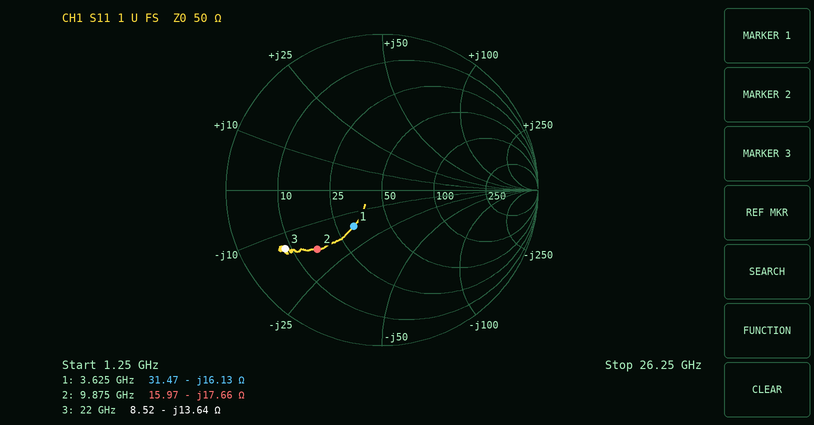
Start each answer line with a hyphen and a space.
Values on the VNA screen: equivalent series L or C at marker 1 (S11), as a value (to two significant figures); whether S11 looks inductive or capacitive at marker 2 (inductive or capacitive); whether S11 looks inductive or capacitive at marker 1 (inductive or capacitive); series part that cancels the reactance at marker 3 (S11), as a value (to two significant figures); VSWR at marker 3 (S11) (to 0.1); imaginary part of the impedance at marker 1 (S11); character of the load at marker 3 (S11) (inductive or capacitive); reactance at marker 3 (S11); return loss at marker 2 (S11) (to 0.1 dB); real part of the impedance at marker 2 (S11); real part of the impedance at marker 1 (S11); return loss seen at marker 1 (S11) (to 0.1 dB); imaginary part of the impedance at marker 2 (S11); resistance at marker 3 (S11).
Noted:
- 2.7 pF
- capacitive
- capacitive
- 99 pH
- 6.3
- -16.13 Ω
- capacitive
- -13.64 Ω
- 5.0 dB
- 15.97 Ω
- 31.47 Ω
- 10.6 dB
- -17.66 Ω
- 8.52 Ω
